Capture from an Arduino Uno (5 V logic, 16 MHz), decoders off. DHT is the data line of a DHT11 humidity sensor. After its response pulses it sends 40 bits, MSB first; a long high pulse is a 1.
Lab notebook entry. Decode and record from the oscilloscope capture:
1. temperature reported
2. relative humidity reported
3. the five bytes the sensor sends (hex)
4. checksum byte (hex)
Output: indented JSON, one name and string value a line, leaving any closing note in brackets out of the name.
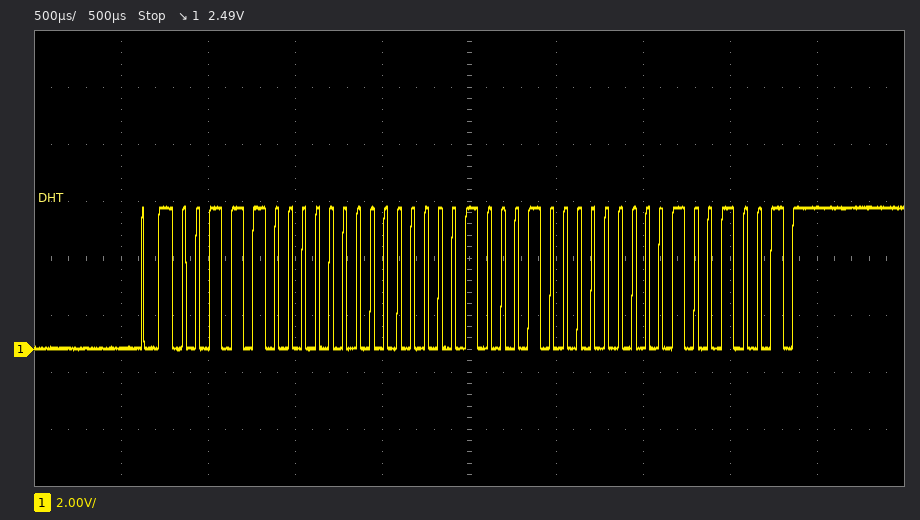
{
  "temperature reported": "17.0 °C",
  "relative humidity reported": "56 %",
  "the five bytes the sensor sends": "38 00 11 00 49",
  "checksum byte": "0x49"
}
